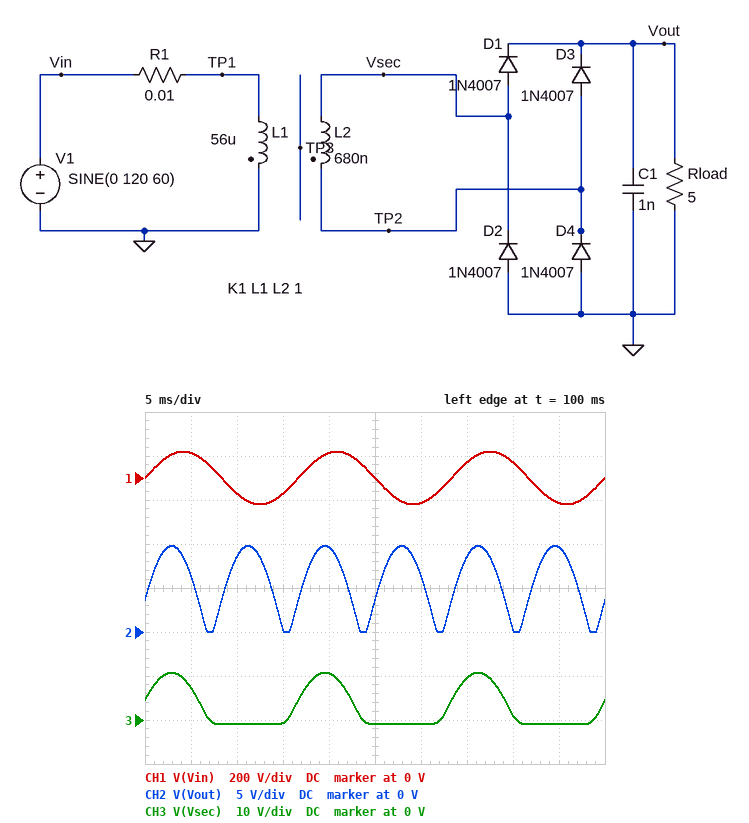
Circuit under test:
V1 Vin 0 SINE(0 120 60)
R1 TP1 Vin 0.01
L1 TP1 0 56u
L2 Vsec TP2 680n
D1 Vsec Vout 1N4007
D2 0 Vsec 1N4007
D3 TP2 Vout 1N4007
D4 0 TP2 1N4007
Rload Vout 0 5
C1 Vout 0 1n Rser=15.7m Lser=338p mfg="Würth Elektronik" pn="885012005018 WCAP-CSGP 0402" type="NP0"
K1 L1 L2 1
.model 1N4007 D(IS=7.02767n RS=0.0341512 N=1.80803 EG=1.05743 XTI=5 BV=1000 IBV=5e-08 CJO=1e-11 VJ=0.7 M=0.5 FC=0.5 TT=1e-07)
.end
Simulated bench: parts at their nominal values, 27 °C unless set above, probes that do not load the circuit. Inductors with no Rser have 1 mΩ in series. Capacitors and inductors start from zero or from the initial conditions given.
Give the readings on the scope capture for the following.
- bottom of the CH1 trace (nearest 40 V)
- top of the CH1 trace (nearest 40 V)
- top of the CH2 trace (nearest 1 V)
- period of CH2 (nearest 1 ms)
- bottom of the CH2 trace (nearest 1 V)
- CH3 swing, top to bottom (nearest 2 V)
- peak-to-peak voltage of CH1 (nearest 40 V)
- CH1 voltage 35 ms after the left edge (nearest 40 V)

-120 V
120 V
10 V
8 ms
0 V
12 V
240 V
80 V
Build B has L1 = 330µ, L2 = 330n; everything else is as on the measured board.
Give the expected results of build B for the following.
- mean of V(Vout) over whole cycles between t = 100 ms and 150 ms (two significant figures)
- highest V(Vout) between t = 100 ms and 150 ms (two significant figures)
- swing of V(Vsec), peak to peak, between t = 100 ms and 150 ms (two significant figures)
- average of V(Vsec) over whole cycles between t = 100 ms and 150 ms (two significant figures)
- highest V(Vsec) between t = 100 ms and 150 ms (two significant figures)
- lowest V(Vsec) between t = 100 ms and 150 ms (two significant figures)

1.0 V
2.1 V
3.8 V
500 mV
2.9 V
-850 mV
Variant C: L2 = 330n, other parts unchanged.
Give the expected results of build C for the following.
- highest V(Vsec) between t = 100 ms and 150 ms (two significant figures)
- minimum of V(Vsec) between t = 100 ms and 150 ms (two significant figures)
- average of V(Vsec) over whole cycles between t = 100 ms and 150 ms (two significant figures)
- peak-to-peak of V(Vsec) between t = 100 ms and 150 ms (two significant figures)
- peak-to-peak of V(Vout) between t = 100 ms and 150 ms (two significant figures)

7.2 V
-930 mV
1.8 V
8.2 V
6.3 V
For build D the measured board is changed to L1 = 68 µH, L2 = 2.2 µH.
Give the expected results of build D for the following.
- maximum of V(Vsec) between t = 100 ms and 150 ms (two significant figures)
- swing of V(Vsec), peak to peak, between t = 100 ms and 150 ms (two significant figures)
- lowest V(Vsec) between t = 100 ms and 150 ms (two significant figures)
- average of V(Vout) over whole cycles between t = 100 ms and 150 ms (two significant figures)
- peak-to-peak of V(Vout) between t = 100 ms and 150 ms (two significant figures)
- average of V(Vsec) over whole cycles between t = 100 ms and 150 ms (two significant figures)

19 V
20 V
-1.1 V
11 V
18 V
5.4 V
